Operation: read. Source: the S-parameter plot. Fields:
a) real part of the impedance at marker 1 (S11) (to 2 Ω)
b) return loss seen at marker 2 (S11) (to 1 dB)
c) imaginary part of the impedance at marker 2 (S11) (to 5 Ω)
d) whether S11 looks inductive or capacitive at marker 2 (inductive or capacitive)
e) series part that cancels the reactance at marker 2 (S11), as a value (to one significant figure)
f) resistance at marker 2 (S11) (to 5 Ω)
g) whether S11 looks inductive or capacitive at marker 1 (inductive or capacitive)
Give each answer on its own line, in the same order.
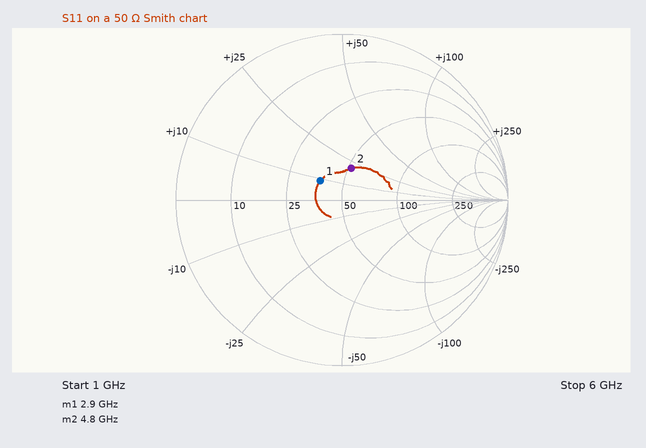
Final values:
38 Ω
14 dB
+20 Ω
inductive
2 pF
50 Ω
inductive
